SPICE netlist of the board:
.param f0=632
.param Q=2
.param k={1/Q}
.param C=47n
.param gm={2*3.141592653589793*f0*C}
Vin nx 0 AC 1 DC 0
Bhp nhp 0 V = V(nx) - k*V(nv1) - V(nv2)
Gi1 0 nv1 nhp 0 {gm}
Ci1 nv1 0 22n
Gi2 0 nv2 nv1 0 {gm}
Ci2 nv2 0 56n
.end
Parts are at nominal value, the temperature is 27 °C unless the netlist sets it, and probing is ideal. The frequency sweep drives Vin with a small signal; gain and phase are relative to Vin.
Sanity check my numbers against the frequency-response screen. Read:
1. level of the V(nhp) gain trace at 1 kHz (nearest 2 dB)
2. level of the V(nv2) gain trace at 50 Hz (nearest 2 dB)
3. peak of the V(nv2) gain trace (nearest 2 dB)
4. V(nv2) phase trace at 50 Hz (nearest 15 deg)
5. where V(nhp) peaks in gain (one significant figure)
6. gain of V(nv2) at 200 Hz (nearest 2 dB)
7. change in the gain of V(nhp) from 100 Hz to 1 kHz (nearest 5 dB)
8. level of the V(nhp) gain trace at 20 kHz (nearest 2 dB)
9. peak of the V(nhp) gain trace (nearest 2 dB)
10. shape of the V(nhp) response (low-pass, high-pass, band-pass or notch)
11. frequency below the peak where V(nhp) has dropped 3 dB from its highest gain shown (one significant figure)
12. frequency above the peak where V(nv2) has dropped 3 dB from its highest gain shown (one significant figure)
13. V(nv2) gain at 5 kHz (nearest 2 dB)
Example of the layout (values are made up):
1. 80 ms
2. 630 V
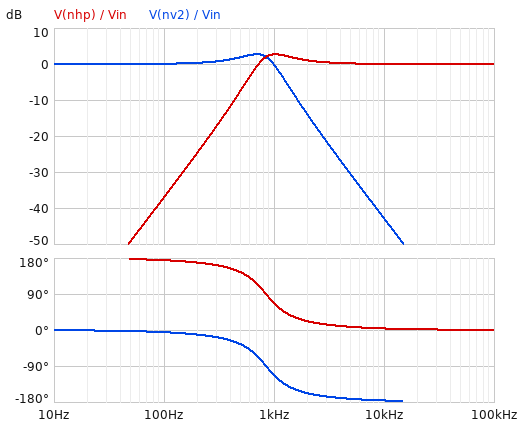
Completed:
1. 2 dB
2. 0 dB
3. 2 dB
4. 0 deg
5. 1 kHz
6. 0 dB
7. 40 dB
8. 0 dB
9. 2 dB
10. high-pass
11. 700 Hz
12. 1 kHz
13. -30 dB
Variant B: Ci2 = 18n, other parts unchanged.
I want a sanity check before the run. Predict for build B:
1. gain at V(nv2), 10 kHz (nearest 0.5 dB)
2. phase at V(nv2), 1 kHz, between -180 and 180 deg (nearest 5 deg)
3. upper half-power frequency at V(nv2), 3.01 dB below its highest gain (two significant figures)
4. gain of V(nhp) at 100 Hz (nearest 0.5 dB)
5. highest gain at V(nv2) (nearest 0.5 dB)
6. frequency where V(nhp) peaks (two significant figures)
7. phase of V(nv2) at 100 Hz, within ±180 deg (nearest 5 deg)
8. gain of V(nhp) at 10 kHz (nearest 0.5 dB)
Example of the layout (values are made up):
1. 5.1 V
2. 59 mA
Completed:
1. -33.0 dB
2. -30 deg
3. 1.7 kHz
4. -47.0 dB
5. 7.0 dB
6. 1.6 kHz
7. 0 deg
8. 0 dB
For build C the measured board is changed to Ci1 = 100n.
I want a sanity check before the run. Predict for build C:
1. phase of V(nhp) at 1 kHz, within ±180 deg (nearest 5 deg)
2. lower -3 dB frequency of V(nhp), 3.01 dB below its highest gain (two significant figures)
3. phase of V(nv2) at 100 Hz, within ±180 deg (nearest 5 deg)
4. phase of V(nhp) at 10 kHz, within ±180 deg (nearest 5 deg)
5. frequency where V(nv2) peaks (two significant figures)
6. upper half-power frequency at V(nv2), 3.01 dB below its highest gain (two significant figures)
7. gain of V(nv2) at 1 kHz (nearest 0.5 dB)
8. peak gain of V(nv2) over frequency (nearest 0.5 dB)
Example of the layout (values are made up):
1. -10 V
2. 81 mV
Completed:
1. 10 deg
2. 350 Hz
3. -5 deg
4. 0 deg
5. 380 Hz
6. 450 Hz
7. -14.5 dB
8. 8.5 dB
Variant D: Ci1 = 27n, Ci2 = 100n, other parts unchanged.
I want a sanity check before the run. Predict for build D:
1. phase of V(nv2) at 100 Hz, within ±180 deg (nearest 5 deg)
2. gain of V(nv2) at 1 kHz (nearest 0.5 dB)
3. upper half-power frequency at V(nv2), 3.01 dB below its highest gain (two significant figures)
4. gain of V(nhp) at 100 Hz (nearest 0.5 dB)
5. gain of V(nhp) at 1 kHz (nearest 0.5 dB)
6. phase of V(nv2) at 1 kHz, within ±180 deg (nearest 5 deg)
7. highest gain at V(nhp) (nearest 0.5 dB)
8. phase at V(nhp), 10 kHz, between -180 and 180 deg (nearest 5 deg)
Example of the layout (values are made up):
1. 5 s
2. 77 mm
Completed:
1. -10 deg
2. -8.5 dB
3. 670 Hz
4. -30.0 dB
5. 1.0 dB
6. -140 deg
7. 1.5 dB
8. 5 deg
